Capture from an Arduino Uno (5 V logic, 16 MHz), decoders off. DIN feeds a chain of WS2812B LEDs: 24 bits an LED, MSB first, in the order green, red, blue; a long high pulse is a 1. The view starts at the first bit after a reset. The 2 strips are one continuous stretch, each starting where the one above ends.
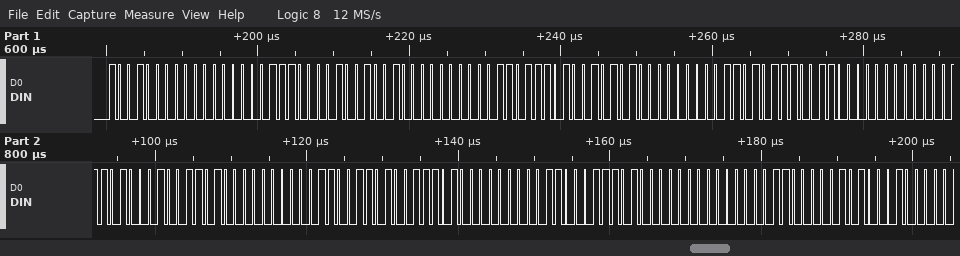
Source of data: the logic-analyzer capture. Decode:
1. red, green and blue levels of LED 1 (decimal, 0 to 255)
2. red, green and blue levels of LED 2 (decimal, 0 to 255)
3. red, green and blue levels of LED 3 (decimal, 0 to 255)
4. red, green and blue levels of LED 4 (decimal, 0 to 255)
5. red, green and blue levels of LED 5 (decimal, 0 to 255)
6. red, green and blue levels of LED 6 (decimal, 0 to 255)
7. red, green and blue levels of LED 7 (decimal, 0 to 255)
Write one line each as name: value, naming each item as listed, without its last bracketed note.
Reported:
red, green and blue levels of LED 1: 0, 144, 112
red, green and blue levels of LED 2: 0, 146, 110
red, green and blue levels of LED 3: 0, 149, 107
red, green and blue levels of LED 4: 0, 152, 104
red, green and blue levels of LED 5: 0, 154, 102
red, green and blue levels of LED 6: 0, 157, 99
red, green and blue levels of LED 7: 0, 160, 96
